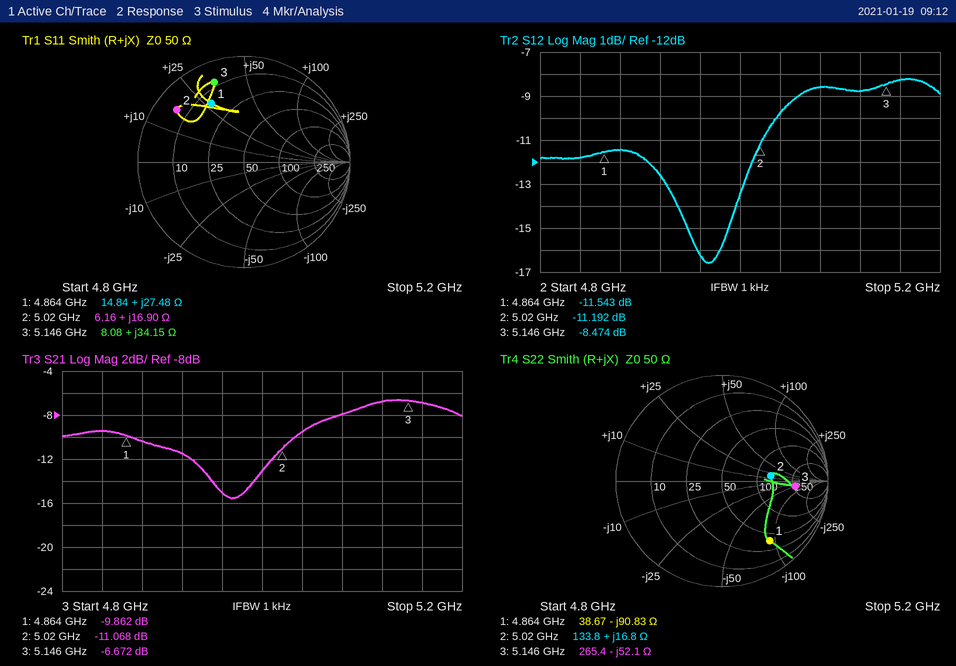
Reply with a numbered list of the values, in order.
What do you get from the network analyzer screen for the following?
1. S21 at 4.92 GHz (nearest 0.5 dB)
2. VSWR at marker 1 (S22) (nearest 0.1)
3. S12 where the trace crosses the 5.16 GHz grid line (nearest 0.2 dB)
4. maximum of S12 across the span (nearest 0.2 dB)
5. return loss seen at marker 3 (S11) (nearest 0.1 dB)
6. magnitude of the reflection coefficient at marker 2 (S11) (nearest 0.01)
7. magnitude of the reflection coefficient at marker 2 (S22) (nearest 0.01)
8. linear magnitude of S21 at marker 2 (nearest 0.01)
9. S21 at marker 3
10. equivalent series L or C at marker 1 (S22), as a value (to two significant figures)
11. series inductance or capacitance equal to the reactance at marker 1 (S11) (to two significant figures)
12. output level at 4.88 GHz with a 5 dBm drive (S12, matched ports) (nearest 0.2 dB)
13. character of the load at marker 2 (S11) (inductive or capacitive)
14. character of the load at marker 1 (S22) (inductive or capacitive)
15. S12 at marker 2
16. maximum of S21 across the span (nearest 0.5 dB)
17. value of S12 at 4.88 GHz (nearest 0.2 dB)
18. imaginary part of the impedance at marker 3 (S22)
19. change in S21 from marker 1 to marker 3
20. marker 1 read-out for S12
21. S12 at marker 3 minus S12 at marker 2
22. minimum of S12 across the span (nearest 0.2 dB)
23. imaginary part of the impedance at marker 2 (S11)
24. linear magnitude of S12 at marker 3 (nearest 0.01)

1. -11.5 dB
2. 6.2
3. -8.2 dB
4. -8.2 dB
5. 1.9 dB
6. 0.80
7. 0.46
8. 0.28
9. -6.672 dB
10. 360 fF
11. 900 pH
12. -6.4 dBm
13. inductive
14. capacitive
15. -11.192 dB
16. -6.5 dB
17. -11.4 dB
18. -52.1 Ω
19. 3.190 dB
20. -11.543 dB
21. 2.718 dB
22. -16.6 dB
23. +16.90 Ω
24. 0.38
